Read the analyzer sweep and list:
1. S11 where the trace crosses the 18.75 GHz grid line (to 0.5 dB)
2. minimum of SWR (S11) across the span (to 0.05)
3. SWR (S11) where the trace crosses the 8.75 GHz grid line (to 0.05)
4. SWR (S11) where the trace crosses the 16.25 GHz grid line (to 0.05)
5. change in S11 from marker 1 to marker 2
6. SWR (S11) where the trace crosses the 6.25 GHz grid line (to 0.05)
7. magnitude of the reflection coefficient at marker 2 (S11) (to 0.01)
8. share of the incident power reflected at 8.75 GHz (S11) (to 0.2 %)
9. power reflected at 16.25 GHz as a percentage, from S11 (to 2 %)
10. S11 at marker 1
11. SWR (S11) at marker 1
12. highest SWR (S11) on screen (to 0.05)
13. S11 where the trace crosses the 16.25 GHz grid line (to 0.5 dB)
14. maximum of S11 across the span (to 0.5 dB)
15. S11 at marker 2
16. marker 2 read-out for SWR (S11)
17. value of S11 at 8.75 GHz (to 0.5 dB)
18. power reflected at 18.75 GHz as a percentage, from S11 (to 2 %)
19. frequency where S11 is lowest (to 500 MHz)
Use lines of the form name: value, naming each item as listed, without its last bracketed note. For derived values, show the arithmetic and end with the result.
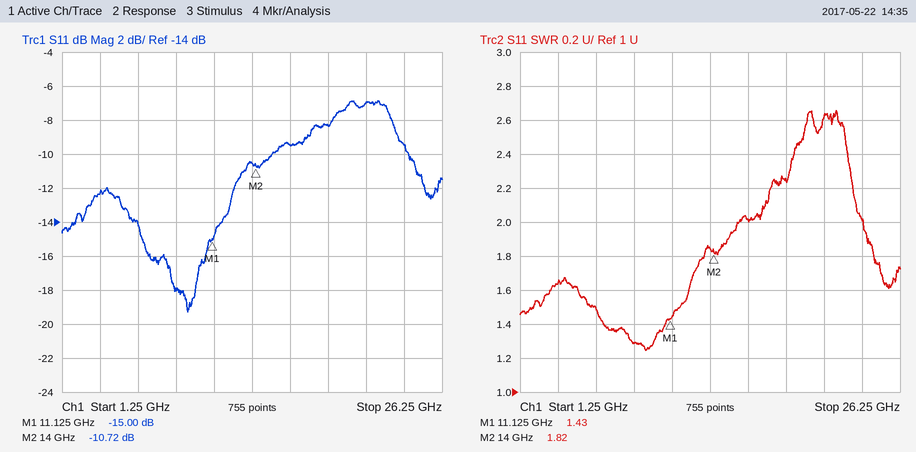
S11 where the trace crosses the 18.75 GHz grid line: -8.5 dB
minimum of SWR (S11) across the span: 1.25
SWR (S11) where the trace crosses the 8.75 GHz grid line: 1.30
SWR (S11) where the trace crosses the 16.25 GHz grid line: 2.00
change in S11 from marker 1 to marker 2: -10.72 − (-15) = 4.28 dB
SWR (S11) where the trace crosses the 6.25 GHz grid line: 1.50
magnitude of the reflection coefficient at marker 2 (S11): 10^(-10.72/20) ≈ 0.29
share of the incident power reflected at 8.75 GHz (S11): 10^(-18/10) ≈ 1.6 %
power reflected at 16.25 GHz as a percentage, from S11: 10^(-9.5/10) ≈ 11.2 %, so 12 % to the nearest 2 %
S11 at marker 1: -15.00 dB
SWR (S11) at marker 1: 1.43
highest SWR (S11) on screen: 2.65
S11 where the trace crosses the 16.25 GHz grid line: -9.5 dB
maximum of S11 across the span: -7.0 dB
S11 at marker 2: -10.72 dB
marker 2 read-out for SWR: 1.82
value of S11 at 8.75 GHz: -18.0 dB
power reflected at 18.75 GHz as a percentage, from S11: 10^(-8.5/10) ≈ 14 %
frequency where S11 is lowest: 9.5 GHz
